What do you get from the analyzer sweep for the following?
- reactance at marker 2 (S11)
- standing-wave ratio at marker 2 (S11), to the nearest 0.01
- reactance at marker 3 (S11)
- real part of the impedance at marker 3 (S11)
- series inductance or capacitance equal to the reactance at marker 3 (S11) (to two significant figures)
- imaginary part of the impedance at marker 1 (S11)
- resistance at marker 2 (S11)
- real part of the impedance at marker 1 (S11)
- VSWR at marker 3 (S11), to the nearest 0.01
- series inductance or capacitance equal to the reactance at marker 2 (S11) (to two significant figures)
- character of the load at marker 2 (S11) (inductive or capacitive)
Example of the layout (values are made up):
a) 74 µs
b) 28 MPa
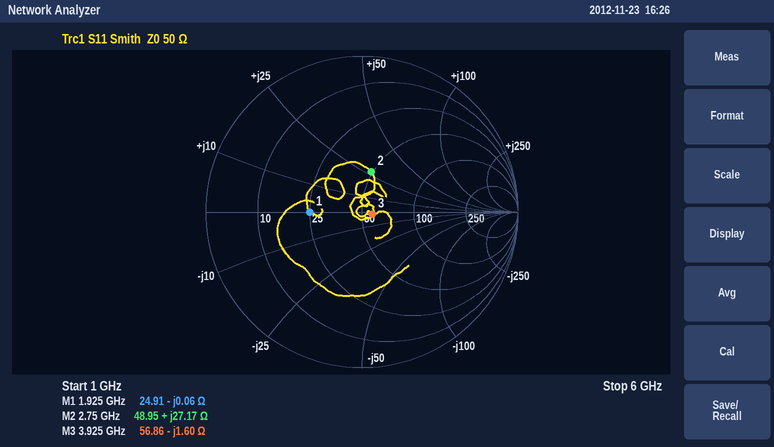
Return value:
a) +27.17 Ω
b) 1.72
c) -1.60 Ω
d) 56.86 Ω
e) 25 pF
f) -0.06 Ω
g) 48.95 Ω
h) 24.91 Ω
i) 1.14
j) 1.6 nH
k) inductive
